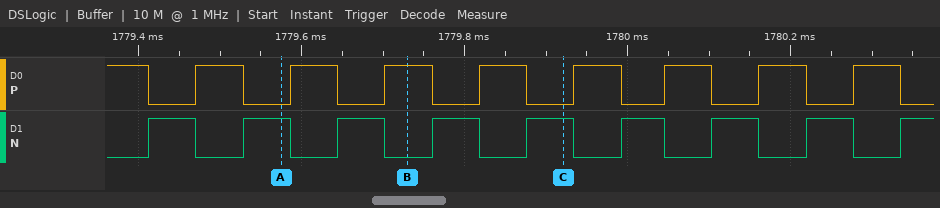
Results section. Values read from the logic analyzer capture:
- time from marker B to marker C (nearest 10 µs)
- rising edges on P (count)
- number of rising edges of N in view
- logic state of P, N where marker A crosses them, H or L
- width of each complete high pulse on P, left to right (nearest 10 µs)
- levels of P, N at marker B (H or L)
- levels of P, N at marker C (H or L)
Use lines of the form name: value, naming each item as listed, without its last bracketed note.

time from marker B to marker C: 190 µs
rising edges on P: 8
number of rising edges of N in view: 9
logic state of P, N where marker A crosses them, H or L: P=L, N=H
width of each complete high pulse on P, left to right: 60 µs, 60 µs, 60 µs, 60 µs, 60 µs, 60 µs, 60 µs, 60 µs
levels of P, N at marker B: P=H, N=L
levels of P, N at marker C: P=L, N=H
